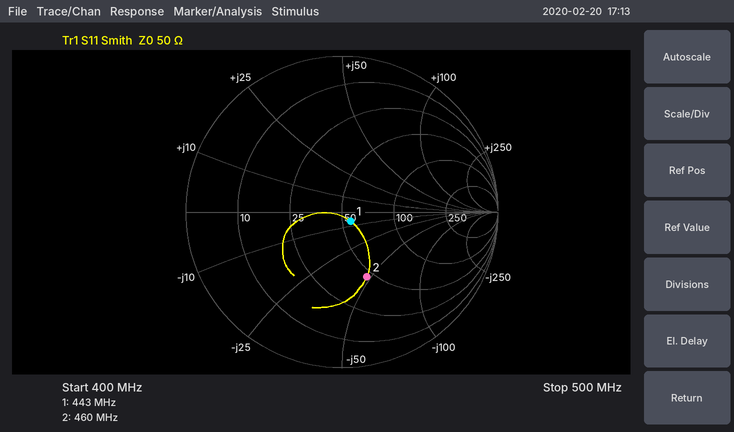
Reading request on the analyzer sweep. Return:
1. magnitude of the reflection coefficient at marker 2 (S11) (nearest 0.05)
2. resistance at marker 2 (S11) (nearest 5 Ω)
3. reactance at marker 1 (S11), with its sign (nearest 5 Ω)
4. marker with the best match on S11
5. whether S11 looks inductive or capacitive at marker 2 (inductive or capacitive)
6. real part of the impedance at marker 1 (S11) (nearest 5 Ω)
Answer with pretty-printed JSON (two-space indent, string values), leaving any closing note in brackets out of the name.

{
  "magnitude of the reflection coefficient at marker 2 (S11)": "0.45",
  "resistance at marker 2 (S11)": "45 Ω",
  "reactance at marker 1 (S11), with its sign": "-5 Ω",
  "marker with the best match on S11": "marker 1",
  "whether S11 looks inductive or capacitive at marker 2": "capacitive",
  "real part of the impedance at marker 1 (S11)": "55 Ω"
}
